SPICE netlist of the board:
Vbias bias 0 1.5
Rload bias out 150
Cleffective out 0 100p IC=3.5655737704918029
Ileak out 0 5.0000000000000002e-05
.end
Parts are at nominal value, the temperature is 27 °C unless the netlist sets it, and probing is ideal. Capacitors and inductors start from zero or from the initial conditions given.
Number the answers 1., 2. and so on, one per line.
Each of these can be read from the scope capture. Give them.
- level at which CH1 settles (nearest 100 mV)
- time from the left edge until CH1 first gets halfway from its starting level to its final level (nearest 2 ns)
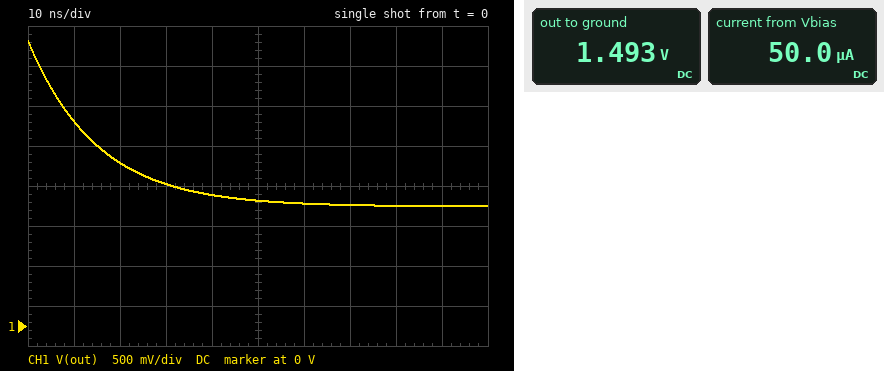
1. 1.5 V
2. 10 ns
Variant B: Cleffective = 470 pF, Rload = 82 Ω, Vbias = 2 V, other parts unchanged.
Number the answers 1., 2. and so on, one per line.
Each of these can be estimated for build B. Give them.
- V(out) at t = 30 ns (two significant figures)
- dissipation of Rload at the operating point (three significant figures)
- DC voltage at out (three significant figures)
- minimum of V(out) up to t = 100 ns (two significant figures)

1. 2.7 V
2. 205 nW
3. 2.00 V
4. 2.1 V
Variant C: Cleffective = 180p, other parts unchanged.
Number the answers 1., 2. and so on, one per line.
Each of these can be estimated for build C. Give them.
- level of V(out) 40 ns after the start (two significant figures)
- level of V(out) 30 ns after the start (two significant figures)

1. 2.0 V
2. 2.2 V
